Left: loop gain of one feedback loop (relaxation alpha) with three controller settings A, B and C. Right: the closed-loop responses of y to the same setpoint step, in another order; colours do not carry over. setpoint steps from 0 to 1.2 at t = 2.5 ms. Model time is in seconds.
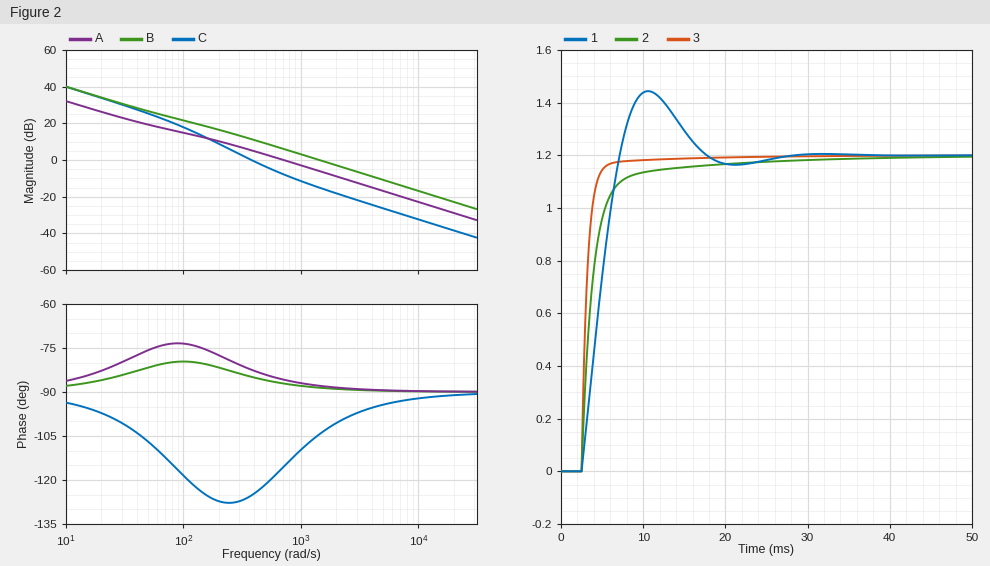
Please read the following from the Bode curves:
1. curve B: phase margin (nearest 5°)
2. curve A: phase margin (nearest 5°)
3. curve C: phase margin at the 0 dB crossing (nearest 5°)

90°
95°
55°
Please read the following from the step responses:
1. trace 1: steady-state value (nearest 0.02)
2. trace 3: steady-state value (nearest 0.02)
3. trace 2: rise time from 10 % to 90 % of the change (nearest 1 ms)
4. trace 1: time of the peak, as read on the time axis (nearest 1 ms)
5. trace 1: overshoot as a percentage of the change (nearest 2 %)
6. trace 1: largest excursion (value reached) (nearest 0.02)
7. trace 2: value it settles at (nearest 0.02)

1.20
1.20
4 ms
11 ms
20 %
1.44
1.20
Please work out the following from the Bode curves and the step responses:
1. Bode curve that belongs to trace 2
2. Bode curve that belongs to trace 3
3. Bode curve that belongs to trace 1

A
B
C
